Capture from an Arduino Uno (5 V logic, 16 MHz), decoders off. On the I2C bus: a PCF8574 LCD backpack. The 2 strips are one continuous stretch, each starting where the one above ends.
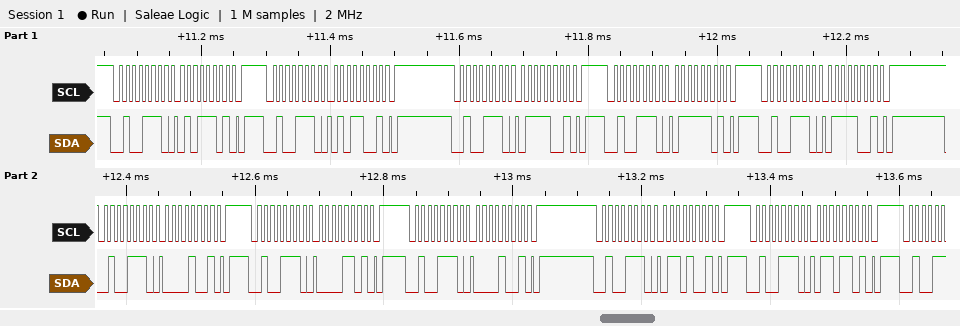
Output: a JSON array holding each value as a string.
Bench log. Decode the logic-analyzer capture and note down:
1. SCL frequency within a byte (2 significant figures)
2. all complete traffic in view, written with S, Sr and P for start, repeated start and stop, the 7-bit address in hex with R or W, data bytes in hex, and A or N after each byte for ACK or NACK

["100 kHz", "S 27W A 5D A P S 27W A 59 A P S 27W A 79 A P S 27W A 7D A P S 27W A 79 A P S 27W A 09 A P S 27W A 0D A P S 27W A 09 A P S 27W A 69 A P S 27W A 6D A P"]
